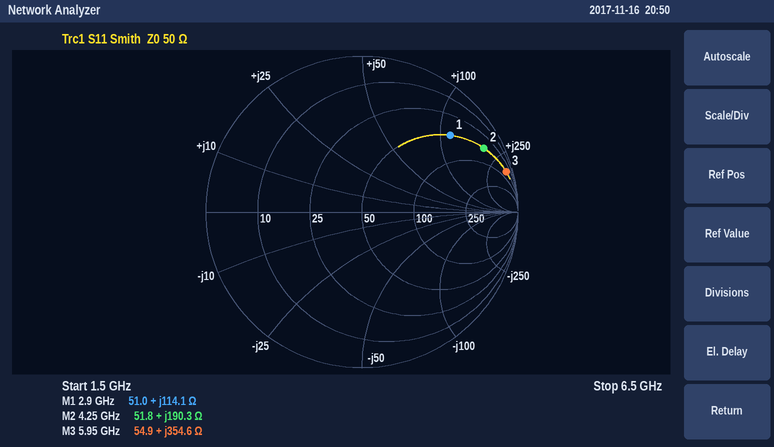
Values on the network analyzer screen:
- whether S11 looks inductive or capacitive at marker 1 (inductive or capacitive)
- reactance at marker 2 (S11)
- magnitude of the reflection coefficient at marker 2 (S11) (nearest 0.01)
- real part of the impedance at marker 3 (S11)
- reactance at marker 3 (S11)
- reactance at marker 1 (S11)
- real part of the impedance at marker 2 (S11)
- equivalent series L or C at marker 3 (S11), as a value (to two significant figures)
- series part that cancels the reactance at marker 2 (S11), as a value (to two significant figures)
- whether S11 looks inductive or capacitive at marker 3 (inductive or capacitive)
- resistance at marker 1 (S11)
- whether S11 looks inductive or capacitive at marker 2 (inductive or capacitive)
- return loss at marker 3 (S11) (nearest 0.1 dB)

inductive
+190.3 Ω
0.88
54.9 Ω
+354.6 Ω
+114.1 Ω
51.8 Ω
9.5 nH
200 fF
inductive
51.0 Ω
inductive
0.4 dB
